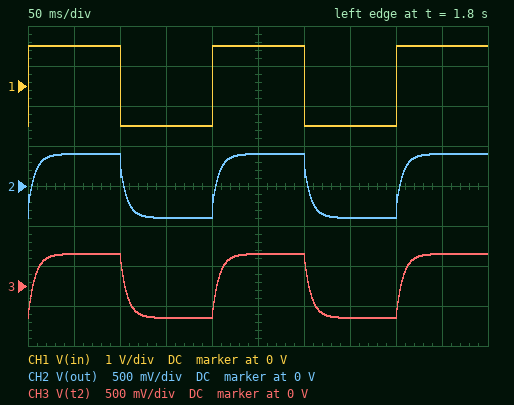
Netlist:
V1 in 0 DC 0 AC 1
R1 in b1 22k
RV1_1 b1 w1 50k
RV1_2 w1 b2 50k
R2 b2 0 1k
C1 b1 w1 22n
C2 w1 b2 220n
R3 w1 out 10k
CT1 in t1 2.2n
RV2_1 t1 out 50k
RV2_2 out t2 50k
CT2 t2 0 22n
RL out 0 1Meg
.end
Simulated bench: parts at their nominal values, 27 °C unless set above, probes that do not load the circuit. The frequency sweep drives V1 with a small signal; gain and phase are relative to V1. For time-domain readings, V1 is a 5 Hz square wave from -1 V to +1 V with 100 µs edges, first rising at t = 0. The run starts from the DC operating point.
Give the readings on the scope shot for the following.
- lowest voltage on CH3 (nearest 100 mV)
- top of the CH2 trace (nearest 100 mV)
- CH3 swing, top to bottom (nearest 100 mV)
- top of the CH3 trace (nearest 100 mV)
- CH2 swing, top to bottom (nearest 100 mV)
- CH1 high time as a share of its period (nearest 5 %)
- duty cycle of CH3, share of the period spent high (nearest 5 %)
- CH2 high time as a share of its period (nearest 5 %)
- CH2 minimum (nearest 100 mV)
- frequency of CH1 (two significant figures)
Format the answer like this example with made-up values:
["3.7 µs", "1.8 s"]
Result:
["-400 mV", "400 mV", "800 mV", "400 mV", "800 mV", "50 %", "50 %", "50 %", "-400 mV", "5.0 Hz"]
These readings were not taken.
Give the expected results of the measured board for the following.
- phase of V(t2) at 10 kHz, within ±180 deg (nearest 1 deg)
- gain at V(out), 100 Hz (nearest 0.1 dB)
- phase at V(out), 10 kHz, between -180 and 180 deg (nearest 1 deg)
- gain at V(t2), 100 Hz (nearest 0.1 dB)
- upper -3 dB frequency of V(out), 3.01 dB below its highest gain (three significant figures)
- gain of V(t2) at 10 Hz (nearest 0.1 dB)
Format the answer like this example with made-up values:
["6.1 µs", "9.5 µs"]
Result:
["-84 deg", "-20.6 dB", "5 deg", "-22.3 dB", "21.6 Hz", "-8.9 dB"]
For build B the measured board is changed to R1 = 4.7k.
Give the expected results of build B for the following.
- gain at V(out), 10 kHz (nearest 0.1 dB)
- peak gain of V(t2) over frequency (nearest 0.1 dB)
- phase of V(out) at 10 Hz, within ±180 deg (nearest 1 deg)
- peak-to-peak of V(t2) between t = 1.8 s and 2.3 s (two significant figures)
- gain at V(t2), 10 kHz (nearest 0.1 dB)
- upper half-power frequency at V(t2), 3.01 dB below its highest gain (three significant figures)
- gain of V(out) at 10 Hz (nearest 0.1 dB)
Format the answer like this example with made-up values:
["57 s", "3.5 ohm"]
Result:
["-11.4 dB", "-6.6 dB", "-19 deg", "930 mV", "-48.2 dB", "23.1 Hz", "-7.4 dB"]
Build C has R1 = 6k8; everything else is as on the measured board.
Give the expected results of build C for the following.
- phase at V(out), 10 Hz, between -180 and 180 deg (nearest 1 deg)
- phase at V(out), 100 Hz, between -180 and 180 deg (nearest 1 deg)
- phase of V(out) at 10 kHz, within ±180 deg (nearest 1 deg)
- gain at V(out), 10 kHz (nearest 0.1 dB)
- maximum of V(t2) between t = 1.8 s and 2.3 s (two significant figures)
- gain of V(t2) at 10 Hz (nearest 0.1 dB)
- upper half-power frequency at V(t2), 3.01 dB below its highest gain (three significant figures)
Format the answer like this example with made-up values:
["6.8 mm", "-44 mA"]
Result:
["-19 deg", "-35 deg", "4 deg", "-12.5 dB", "460 mV", "-7.6 dB", "22.8 Hz"]
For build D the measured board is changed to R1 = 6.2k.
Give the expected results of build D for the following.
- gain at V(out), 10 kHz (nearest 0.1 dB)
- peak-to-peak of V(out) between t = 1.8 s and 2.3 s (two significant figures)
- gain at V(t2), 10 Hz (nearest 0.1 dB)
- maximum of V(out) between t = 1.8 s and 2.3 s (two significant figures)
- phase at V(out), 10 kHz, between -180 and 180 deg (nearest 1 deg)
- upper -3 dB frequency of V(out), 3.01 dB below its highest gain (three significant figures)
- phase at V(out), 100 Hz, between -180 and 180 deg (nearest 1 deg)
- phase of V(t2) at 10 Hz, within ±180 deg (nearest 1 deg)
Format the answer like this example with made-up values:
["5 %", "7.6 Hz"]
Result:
["-12.2 dB", "920 mV", "-7.5 dB", "460 mV", "4 deg", "23.5 Hz", "-35 deg", "-23 deg"]
